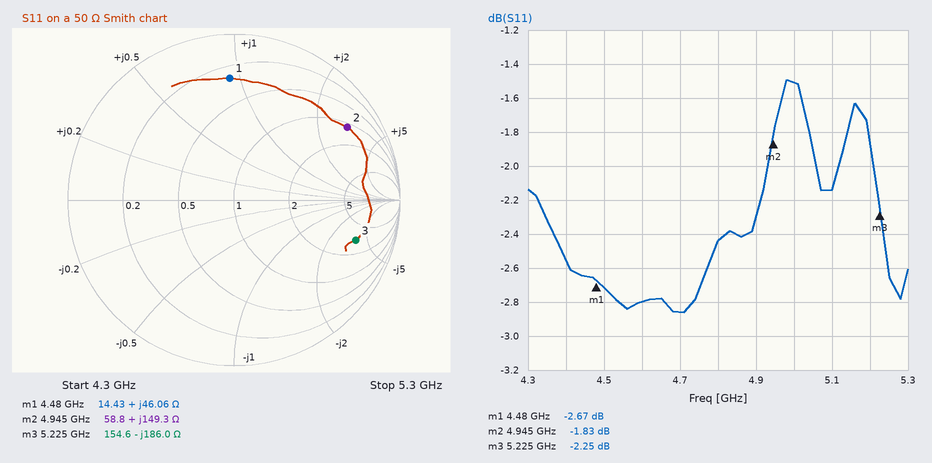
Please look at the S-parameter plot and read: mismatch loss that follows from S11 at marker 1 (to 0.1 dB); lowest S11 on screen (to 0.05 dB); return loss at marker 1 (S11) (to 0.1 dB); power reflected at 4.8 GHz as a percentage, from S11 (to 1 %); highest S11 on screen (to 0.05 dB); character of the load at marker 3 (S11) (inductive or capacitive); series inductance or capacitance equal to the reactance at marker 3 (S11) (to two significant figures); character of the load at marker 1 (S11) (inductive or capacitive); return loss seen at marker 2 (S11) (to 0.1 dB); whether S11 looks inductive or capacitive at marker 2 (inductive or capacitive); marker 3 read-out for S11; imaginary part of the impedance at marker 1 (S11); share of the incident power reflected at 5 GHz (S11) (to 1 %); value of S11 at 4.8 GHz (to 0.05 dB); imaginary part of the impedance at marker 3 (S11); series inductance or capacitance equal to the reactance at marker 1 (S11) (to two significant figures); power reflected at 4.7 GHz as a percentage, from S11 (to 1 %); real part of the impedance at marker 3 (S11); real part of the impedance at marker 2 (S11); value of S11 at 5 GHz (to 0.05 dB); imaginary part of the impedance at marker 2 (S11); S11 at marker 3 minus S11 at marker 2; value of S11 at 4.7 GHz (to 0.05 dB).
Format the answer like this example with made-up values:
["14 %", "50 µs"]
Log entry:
["3.4 dB", "-2.85 dB", "2.7 dB", "57 %", "-1.50 dB", "capacitive", "160 fF", "inductive", "1.8 dB", "inductive", "-2.25 dB", "+46.06 Ω", "71 %", "-2.45 dB", "-186.0 Ω", "1.6 nH", "52 %", "154.6 Ω", "58.8 Ω", "-1.50 dB", "+149.3 Ω", "-0.42 dB", "-2.85 dB"]
